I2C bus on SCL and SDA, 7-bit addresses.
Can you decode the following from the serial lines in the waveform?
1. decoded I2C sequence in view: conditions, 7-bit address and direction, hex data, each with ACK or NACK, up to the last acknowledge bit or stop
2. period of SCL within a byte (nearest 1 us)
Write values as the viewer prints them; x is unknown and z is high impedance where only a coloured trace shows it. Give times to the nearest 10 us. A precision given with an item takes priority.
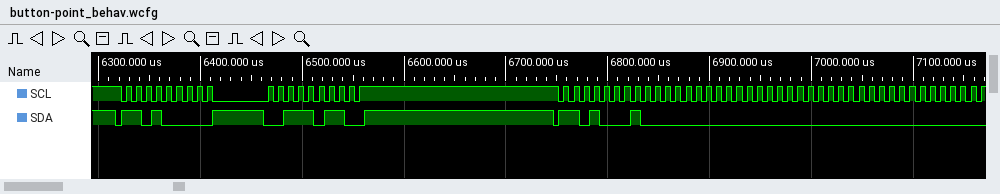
start, address 68 write ACK, 3B ACK, stop, start, address 68 read ACK, 00 ACK, 00 ACK, 00 ACK
10 us
